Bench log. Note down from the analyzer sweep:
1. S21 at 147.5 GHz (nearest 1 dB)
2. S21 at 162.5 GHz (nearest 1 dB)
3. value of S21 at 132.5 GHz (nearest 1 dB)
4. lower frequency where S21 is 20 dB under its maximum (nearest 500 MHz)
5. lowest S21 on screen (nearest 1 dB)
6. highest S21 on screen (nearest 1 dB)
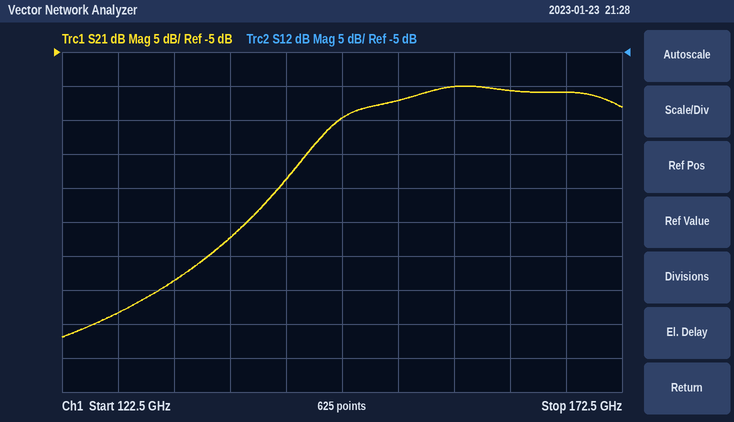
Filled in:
-15 dB
-11 dB
-39 dB
139.0 GHz
-47 dB
-10 dB
